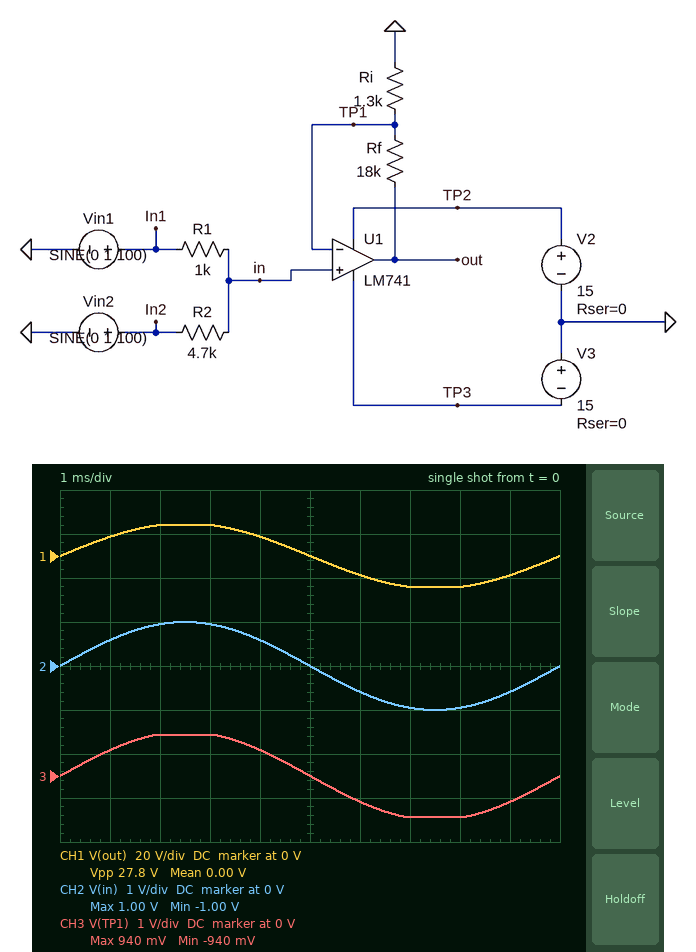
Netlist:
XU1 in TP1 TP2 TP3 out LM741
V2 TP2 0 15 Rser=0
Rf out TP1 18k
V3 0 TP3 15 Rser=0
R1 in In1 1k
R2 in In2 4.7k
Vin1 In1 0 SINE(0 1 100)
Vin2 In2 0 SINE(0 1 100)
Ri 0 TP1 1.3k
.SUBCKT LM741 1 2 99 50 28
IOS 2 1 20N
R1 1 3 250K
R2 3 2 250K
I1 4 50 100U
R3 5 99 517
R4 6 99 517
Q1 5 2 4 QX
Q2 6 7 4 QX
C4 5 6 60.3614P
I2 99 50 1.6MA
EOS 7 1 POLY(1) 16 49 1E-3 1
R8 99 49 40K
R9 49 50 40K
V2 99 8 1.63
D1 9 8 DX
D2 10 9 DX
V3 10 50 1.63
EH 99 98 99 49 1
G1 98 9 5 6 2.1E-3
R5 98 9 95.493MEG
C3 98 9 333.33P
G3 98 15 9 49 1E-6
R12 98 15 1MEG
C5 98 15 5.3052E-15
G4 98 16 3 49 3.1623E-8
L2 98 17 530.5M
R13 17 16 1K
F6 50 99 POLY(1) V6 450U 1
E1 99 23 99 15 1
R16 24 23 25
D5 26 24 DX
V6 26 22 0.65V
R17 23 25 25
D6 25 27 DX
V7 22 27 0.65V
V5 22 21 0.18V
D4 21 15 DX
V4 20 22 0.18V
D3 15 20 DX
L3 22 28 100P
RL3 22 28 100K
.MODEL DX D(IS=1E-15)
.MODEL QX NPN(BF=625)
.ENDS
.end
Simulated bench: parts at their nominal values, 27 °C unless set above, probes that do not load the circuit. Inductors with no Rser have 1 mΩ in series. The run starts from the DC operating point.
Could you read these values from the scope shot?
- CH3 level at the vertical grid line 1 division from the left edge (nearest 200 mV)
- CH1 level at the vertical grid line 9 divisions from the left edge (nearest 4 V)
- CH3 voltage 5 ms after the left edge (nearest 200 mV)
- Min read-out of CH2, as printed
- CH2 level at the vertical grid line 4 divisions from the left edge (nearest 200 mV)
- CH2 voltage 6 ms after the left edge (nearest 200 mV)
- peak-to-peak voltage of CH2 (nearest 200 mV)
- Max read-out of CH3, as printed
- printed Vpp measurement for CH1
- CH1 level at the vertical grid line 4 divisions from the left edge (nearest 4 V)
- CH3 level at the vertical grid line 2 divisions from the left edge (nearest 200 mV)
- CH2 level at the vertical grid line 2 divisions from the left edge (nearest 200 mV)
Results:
600 mV
-8 V
0 V
-1.00 V
600 mV
-600 mV
2.0 V
940 mV
27.8 V
8 V
1.0 V
1.0 V
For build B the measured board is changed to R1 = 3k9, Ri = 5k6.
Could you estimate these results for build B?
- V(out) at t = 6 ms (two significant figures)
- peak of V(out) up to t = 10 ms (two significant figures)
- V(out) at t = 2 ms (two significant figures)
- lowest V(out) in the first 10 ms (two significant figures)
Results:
-2.5 V
4.2 V
4.0 V
-4.2 V
